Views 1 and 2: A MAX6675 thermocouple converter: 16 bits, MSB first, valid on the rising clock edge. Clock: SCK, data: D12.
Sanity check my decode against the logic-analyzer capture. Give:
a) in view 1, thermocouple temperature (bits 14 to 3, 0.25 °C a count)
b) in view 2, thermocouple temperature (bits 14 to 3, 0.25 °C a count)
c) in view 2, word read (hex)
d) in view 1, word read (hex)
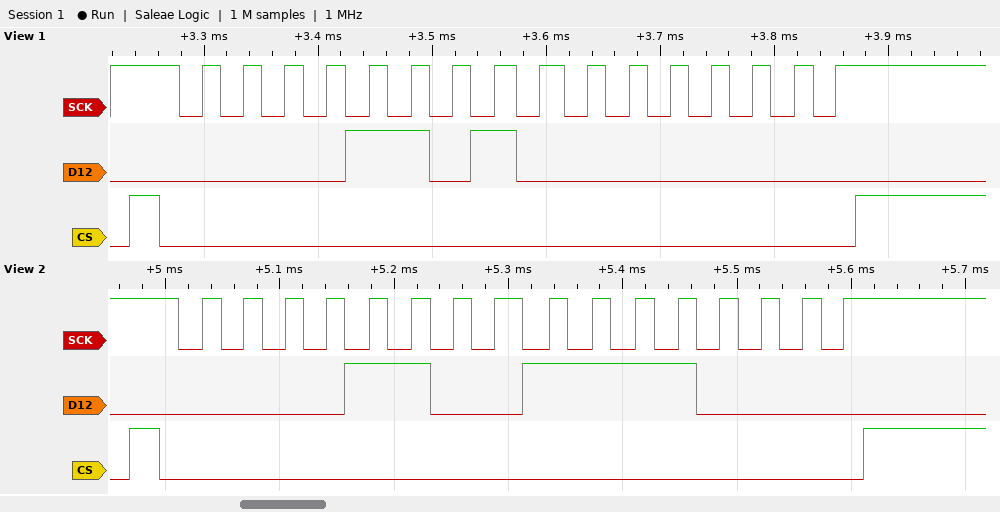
104.00 °C
103.50 °C
0x0CF0
0x0D00
